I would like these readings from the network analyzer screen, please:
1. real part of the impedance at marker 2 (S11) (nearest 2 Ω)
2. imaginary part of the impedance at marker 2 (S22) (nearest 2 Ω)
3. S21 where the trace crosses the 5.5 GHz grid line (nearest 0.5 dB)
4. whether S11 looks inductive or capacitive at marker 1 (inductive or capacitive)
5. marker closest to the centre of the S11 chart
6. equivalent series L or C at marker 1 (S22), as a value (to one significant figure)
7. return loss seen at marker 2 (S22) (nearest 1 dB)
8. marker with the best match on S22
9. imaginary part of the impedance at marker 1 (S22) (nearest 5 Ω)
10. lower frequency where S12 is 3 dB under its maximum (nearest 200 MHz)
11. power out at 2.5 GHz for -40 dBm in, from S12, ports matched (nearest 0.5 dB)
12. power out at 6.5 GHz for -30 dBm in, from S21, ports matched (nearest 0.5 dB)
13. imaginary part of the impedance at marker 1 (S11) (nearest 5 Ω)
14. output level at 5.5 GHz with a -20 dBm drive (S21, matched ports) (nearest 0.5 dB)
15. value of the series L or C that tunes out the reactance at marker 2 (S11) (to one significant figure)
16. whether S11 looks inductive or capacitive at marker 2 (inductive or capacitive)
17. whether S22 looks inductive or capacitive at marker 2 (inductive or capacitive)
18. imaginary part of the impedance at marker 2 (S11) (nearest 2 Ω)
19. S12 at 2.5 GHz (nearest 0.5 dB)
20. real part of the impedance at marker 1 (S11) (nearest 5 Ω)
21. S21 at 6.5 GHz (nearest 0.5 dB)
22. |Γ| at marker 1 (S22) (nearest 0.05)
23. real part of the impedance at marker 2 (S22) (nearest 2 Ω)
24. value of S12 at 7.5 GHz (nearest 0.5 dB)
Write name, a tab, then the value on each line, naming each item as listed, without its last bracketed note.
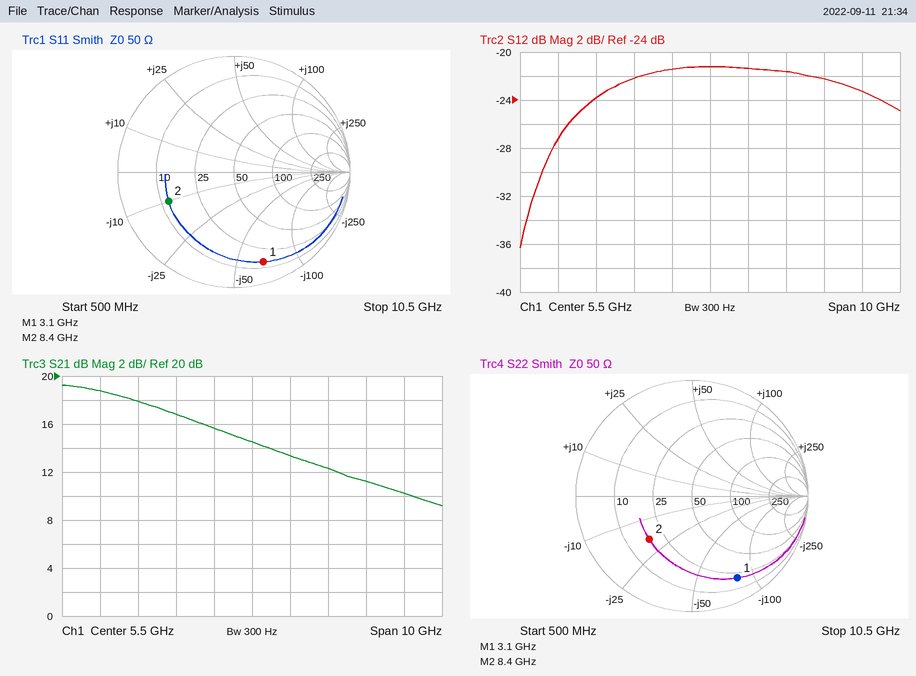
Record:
real part of the impedance at marker 2 (S11)	12 Ω
imaginary part of the impedance at marker 2 (S22)	-18 Ω
S21 where the trace crosses the 5.5 GHz grid line	14.5 dB
whether S11 looks inductive or capacitive at marker 1	capacitive
marker closest to the centre of the S11 chart	marker 2
equivalent series L or C at marker 1 (S22), as a value	600 fF
return loss seen at marker 2 (S22)	6 dB
marker with the best match on S22	marker 2
imaginary part of the impedance at marker 1 (S22)	-80 Ω
lower frequency where S12 is 3 dB under its maximum	2.4 GHz
power out at 2.5 GHz for -40 dBm in, from S12, ports matched	-64.0 dBm
power out at 6.5 GHz for -30 dBm in, from S21, ports matched	-16.5 dBm
imaginary part of the impedance at marker 1 (S11)	-65 Ω
output level at 5.5 GHz with a -20 dBm drive (S21, matched ports)	-5.5 dBm
value of the series L or C that tunes out the reactance at marker 2 (S11)	200 pH
whether S11 looks inductive or capacitive at marker 2	capacitive
whether S22 looks inductive or capacitive at marker 2	capacitive
imaginary part of the impedance at marker 2 (S11)	-10 Ω
S12 at 2.5 GHz	-24.0 dB
real part of the impedance at marker 1 (S11)	15 Ω
S21 at 6.5 GHz	13.5 dB
|Γ| at marker 1 (S22)	0.80
real part of the impedance at marker 2 (S22)	18 Ω
value of S12 at 7.5 GHz	-21.5 dB
